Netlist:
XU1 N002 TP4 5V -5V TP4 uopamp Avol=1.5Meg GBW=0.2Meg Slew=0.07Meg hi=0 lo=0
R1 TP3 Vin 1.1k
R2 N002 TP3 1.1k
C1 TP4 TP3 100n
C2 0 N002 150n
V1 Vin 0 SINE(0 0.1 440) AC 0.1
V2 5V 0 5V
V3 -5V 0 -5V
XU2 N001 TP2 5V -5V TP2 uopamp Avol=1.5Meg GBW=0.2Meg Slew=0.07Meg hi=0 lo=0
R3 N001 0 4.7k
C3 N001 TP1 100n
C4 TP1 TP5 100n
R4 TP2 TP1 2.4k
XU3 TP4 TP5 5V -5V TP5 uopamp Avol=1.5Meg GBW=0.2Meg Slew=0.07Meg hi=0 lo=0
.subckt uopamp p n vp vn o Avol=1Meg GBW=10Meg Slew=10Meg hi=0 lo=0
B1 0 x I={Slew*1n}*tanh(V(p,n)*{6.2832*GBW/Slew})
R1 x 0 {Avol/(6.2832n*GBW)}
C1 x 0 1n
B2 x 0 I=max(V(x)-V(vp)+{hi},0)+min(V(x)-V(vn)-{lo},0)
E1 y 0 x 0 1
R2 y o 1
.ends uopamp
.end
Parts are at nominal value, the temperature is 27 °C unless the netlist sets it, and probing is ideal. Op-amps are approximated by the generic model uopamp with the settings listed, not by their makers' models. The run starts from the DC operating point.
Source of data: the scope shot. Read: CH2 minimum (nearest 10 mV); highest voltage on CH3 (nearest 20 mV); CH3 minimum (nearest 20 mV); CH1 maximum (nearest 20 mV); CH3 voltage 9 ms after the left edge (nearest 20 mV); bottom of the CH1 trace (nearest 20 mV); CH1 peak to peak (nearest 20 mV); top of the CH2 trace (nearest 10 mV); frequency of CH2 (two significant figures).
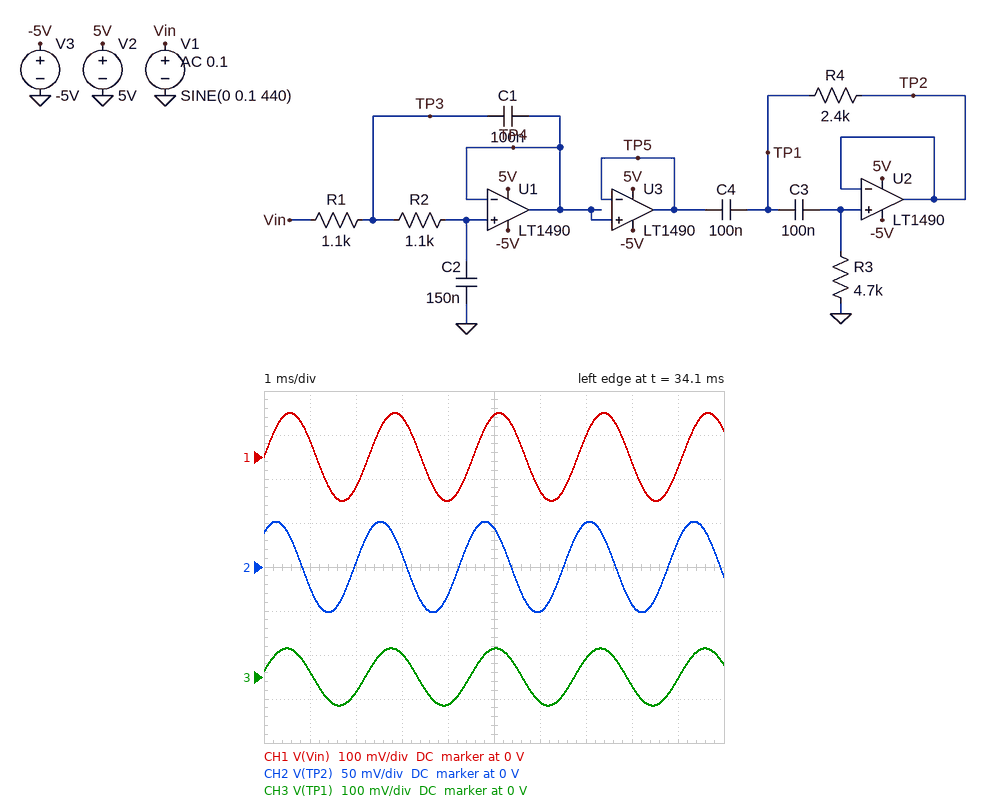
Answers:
-50 mV
60 mV
-60 mV
100 mV
0 V
-100 mV
200 mV
50 mV
440 Hz
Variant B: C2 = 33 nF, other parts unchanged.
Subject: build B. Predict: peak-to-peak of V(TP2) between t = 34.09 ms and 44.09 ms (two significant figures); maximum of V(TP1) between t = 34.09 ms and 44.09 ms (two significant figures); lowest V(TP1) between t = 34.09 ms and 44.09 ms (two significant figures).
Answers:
130 mV
82 mV
-82 mV
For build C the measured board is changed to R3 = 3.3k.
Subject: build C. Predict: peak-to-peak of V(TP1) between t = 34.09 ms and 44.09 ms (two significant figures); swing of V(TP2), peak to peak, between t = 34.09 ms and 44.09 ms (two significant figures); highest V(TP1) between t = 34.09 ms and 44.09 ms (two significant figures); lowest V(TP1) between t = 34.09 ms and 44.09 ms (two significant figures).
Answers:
100 mV
70 mV
52 mV
-52 mV
